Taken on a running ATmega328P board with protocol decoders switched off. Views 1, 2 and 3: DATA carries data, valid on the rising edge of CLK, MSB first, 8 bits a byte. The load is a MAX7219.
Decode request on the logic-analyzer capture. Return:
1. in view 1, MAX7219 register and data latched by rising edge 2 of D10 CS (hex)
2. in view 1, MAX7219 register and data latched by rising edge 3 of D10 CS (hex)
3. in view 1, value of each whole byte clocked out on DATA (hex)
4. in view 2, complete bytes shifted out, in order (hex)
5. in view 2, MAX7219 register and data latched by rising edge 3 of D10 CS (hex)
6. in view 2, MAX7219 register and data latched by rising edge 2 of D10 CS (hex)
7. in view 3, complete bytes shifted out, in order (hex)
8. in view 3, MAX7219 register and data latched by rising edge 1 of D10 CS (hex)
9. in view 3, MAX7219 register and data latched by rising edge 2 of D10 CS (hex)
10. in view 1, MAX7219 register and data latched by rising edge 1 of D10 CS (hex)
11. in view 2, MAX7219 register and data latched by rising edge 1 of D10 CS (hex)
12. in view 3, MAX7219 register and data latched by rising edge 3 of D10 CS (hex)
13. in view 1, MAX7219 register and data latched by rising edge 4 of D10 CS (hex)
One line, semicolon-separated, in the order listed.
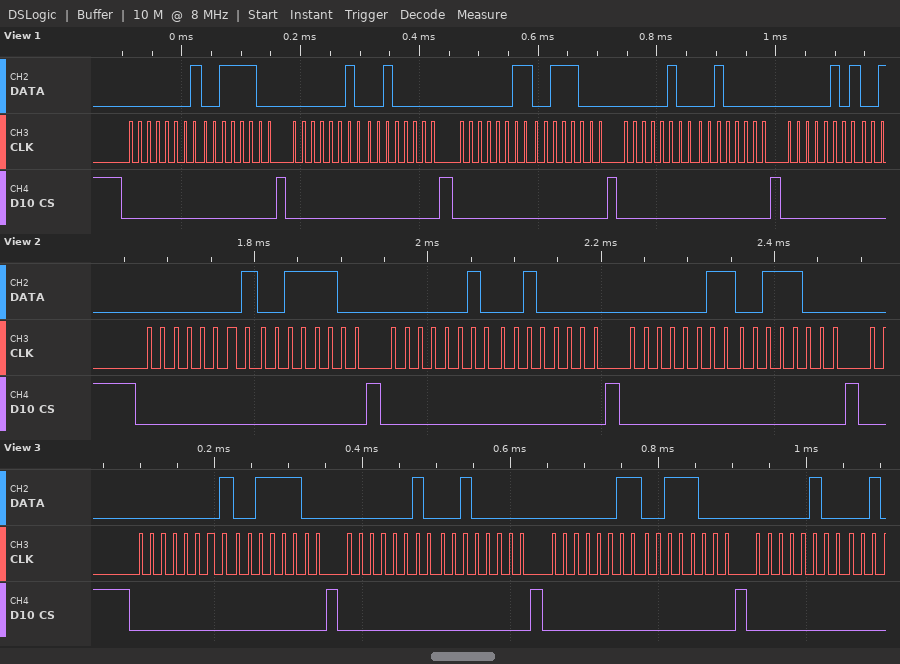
register 0x2, data 0x20; register 0x3, data 0x38; 01 3C 02 20 03 38 04 20 05; 01 3C 02 20 03 38; register 0x3, data 0x38; register 0x2, data 0x20; 0x01 0x3C 0x02 0x20 0x03 0x38 0x04; register 0x1, data 0x3C; register 0x2, data 0x20; register 0x1, data 0x3C; register 0x1, data 0x3C; register 0x3, data 0x38; register 0x4, data 0x20
